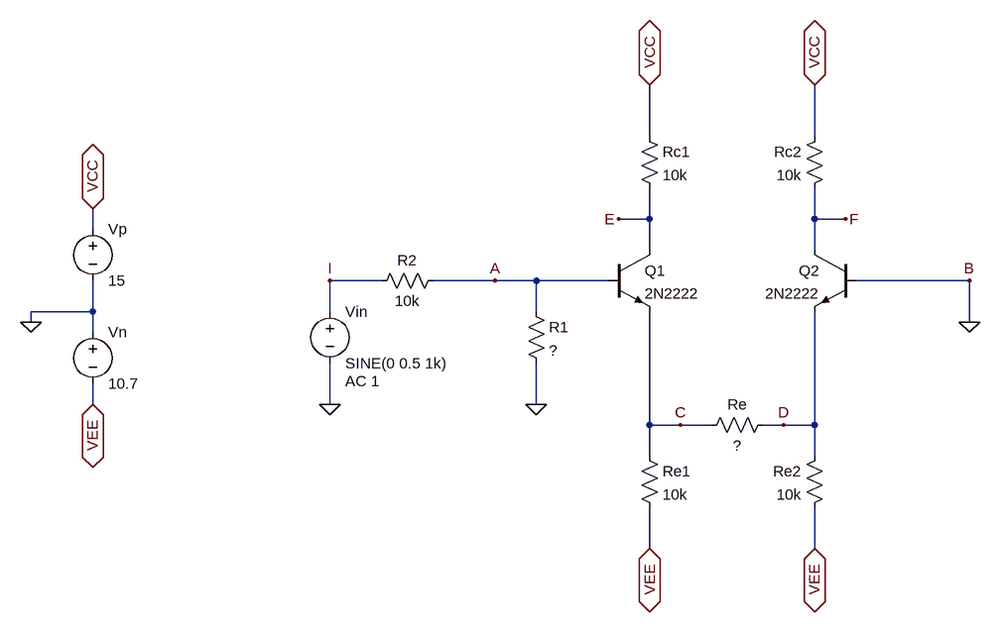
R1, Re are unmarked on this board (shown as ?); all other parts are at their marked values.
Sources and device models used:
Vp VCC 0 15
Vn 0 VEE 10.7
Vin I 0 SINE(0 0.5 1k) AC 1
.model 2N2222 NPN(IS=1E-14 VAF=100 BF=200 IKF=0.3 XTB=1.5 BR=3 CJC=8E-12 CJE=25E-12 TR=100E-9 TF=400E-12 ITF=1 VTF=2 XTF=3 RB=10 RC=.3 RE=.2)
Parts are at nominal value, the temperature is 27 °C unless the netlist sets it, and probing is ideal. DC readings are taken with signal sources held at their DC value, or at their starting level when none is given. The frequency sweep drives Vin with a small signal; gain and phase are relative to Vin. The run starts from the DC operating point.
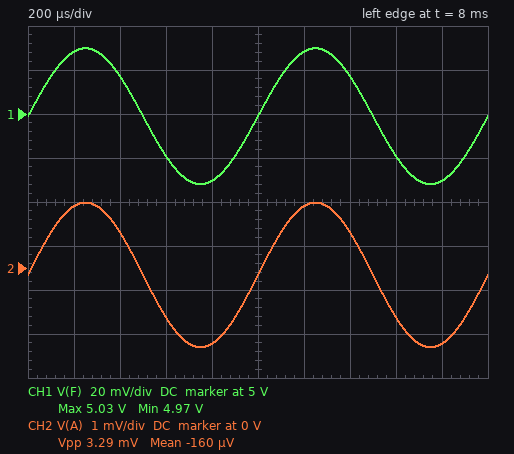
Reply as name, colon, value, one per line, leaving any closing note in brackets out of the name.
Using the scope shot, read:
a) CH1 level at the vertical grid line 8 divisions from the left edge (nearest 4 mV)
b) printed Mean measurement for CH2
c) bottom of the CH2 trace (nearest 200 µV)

CH1 level at the vertical grid line 8 divisions from the left edge: 4.980 V
printed Mean measurement for CH2: -160 µV
bottom of the CH2 trace: -1.8 mV
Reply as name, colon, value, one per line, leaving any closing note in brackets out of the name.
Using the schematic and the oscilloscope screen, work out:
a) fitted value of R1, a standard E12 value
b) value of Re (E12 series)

fitted value of R1, a standard E12 value: 33 Ω
value of Re: 470 Ω
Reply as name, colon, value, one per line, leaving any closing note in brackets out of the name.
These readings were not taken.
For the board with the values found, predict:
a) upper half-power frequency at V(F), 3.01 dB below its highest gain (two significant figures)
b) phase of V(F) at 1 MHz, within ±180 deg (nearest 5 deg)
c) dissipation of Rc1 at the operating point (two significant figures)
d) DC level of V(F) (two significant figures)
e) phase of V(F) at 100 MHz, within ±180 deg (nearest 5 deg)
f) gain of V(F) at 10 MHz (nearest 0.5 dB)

upper half-power frequency at V(F), 3.01 dB below its highest gain: 3.5 MHz
phase of V(F) at 1 MHz, within ±180 deg: -15 deg
dissipation of Rc1 at the operating point: 10 mW
DC level of V(F): 5.0 V
phase of V(F) at 100 MHz, within ±180 deg: -125 deg
gain of V(F) at 10 MHz: -34.0 dB
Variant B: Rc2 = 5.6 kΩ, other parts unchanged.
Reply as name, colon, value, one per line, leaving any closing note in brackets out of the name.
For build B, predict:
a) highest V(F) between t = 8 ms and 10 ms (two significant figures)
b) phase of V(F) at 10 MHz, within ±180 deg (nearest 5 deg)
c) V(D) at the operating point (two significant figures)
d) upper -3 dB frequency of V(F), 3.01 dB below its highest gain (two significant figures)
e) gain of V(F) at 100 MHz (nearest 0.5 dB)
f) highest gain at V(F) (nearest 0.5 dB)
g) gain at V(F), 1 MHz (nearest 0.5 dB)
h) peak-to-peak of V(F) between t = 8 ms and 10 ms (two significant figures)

highest V(F) between t = 8 ms and 10 ms: 9.4 V
phase of V(F) at 10 MHz, within ±180 deg: -55 deg
V(D) at the operating point: -650 mV
upper -3 dB frequency of V(F), 3.01 dB below its highest gain: 7.1 MHz
gain of V(F) at 100 MHz: -54.0 dB
highest gain at V(F): -29.0 dB
gain at V(F), 1 MHz: -29.5 dB
peak-to-peak of V(F) between t = 8 ms and 10 ms: 35 mV
